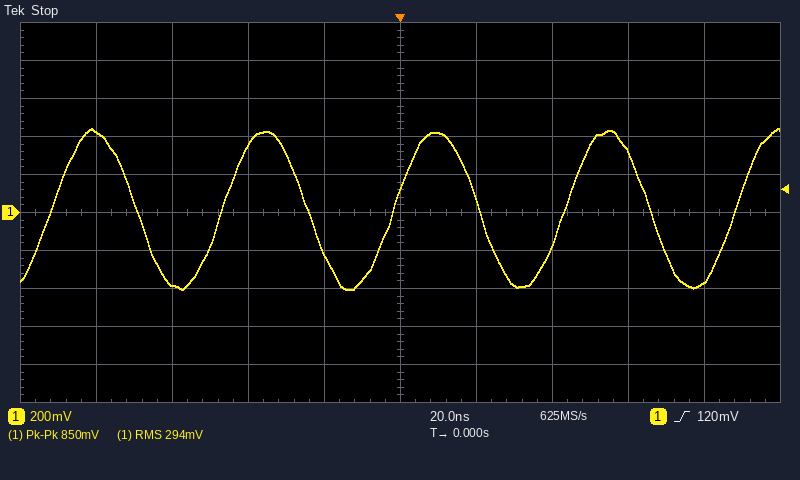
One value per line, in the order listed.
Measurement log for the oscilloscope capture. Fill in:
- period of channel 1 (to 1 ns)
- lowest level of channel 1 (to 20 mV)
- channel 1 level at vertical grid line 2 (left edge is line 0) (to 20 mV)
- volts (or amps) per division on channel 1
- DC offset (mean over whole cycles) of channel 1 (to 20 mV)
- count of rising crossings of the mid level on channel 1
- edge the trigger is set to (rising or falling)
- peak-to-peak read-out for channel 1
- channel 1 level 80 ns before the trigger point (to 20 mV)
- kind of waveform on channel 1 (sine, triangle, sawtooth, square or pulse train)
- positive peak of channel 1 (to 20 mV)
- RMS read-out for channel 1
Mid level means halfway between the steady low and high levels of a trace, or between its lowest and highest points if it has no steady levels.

45 ns
-400 mV
-380 mV
200 mV
20 mV
5
rising
850 mV
420 mV
sine
440 mV
294 mV
